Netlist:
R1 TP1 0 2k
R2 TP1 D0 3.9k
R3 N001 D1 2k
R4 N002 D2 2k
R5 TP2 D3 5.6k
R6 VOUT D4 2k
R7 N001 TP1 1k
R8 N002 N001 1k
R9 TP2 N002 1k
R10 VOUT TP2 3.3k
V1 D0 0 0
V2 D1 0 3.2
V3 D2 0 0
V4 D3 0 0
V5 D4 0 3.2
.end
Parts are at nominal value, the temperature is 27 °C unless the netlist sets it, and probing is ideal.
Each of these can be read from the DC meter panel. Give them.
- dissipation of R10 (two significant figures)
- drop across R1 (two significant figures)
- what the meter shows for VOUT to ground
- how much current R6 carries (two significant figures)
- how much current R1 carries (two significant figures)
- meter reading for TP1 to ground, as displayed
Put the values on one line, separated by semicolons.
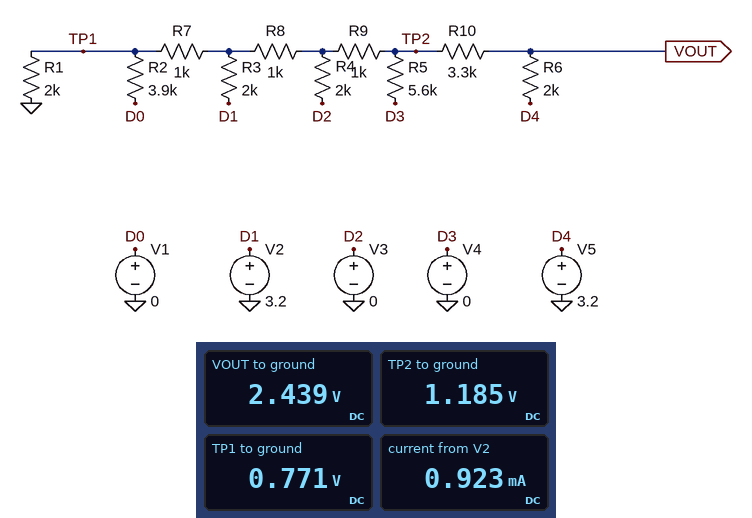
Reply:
480 µW; 770 mV; 2.439 V; 380 µA; 390 µA; 0.771 V
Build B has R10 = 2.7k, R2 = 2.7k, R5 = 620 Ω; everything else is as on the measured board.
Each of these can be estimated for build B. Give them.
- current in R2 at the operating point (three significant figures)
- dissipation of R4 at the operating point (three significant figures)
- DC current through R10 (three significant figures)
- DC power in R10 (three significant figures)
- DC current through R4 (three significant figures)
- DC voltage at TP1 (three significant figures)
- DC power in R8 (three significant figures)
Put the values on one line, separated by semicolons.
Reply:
226 µA; 208 µW; 581 µA; 912 µW; 322 µA; 611 mV; 248 µW
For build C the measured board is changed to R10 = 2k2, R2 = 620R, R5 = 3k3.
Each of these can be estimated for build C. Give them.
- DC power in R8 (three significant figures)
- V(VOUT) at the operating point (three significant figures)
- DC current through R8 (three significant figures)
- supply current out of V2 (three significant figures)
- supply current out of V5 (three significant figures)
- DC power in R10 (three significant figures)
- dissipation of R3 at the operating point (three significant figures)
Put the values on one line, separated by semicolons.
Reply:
66.0 µW; 2.18 V; 257 µA; 1.03 mA; 508 µA; 567 µW; 2.12 mW
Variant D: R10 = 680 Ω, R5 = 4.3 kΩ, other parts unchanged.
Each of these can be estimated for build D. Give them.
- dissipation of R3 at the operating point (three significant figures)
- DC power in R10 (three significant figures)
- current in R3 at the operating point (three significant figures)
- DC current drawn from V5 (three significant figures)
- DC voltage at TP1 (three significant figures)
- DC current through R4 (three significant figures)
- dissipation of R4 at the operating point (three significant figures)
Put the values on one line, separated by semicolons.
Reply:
1.57 mW; 285 µW; 886 µA; 648 µA; 813 mV; 578 µA; 669 µW
